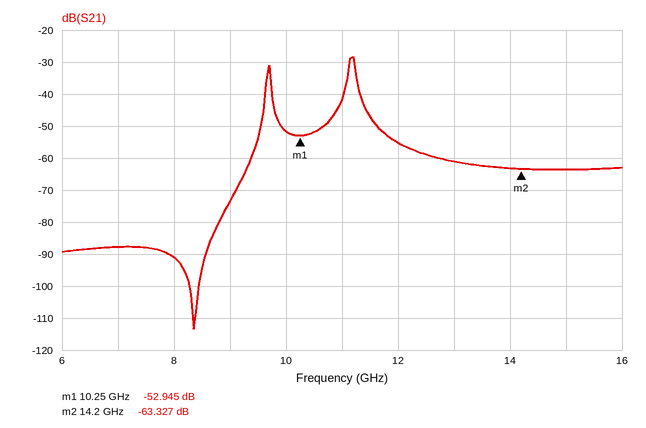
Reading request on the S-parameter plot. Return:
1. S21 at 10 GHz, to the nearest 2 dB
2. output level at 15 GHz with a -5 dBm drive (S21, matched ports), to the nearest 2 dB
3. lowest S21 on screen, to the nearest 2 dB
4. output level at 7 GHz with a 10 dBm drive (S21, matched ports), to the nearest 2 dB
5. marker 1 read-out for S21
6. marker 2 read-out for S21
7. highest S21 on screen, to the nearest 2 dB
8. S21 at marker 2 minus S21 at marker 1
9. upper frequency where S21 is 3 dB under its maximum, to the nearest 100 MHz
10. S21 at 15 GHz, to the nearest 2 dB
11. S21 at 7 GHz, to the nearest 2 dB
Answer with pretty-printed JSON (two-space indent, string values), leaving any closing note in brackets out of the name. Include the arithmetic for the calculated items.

{
  "S21 at 10 GHz, to the nearest 2 dB": "-52 dB",
  "output level at 15 GHz with a -5 dBm drive (S21, matched ports), to the nearest 2 dB": "-5 dBm + (-64 dB) = -68 dBm",
  "lowest S21 on screen, to the nearest 2 dB": "-114 dB",
  "output level at 7 GHz with a 10 dBm drive (S21, matched ports), to the nearest 2 dB": "10 dBm + (-88 dB) = -78 dBm",
  "marker 1 read-out for S21": "-52.945 dB",
  "marker 2 read-out for S21": "-63.327 dB",
  "highest S21 on screen, to the nearest 2 dB": "-28 dB",
  "S21 at marker 2 minus S21 at marker 1": "-63.327 − (-52.945) = -10.382 dB",
  "upper frequency where S21 is 3 dB under its maximum, to the nearest 100 MHz": "11.2 GHz",
  "S21 at 15 GHz, to the nearest 2 dB": "-64 dB",
  "S21 at 7 GHz, to the nearest 2 dB": "-88 dB"
}
